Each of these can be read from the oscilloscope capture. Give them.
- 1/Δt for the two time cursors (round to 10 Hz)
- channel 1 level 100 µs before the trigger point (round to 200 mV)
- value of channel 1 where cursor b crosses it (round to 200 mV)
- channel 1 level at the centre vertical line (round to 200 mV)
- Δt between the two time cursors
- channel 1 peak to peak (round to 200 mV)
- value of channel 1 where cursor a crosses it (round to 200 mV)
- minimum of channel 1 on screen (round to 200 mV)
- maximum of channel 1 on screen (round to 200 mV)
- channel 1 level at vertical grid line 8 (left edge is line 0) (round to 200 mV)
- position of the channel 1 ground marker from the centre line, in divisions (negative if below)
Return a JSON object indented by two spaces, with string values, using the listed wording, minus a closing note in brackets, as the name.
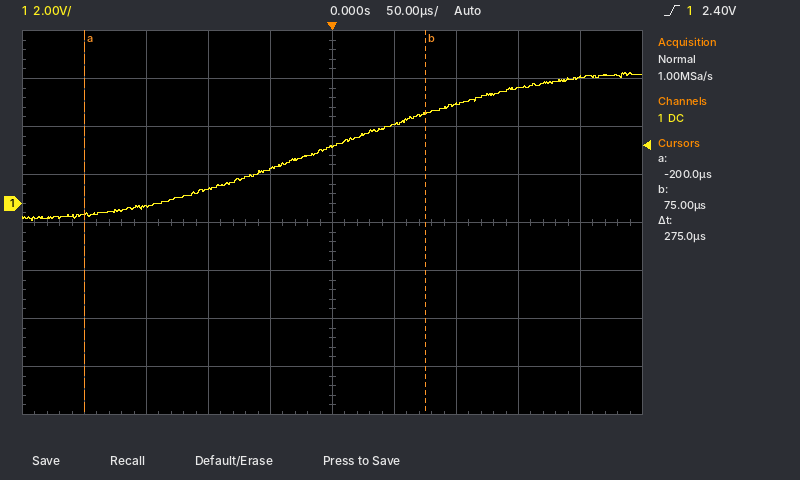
{
  "1/Δt for the two time cursors": "3.64 kHz",
  "channel 1 level 100 µs before the trigger point": "600 mV",
  "value of channel 1 where cursor b crosses it": "3.8 V",
  "channel 1 level at the centre vertical line": "2.4 V",
  "Δt between the two time cursors": "275 µs",
  "channel 1 peak to peak": "6.2 V",
  "value of channel 1 where cursor a crosses it": "-400 mV",
  "minimum of channel 1 on screen": "-800 mV",
  "maximum of channel 1 on screen": "5.4 V",
  "channel 1 level at vertical grid line 8 (left edge is line 0)": "4.8 V",
  "position of the channel 1 ground marker from the centre line, in divisions": "+0.4 div"
}
